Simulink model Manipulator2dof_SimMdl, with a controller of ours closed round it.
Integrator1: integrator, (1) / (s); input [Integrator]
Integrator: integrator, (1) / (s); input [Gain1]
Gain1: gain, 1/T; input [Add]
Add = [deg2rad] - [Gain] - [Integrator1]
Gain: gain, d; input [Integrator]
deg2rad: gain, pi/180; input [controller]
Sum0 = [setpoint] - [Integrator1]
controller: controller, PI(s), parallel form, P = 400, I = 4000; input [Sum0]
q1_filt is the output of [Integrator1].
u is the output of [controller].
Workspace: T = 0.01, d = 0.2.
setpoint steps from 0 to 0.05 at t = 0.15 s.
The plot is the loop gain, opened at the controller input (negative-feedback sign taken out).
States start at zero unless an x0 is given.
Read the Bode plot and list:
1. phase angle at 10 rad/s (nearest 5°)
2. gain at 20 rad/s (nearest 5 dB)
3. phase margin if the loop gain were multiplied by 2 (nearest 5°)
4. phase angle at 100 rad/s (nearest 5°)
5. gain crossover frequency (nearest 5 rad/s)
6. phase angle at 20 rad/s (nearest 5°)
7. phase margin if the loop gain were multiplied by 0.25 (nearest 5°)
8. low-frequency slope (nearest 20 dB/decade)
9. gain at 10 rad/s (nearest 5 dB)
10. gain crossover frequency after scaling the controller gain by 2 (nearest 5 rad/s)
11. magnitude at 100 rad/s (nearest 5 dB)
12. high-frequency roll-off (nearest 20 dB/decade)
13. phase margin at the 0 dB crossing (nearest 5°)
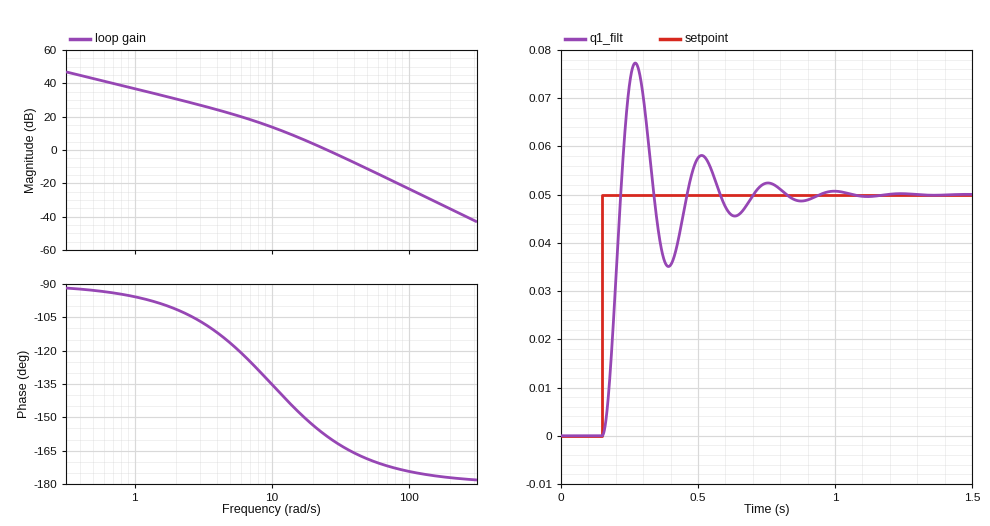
-135°
5 dB
15°
-175°
25 rad/s
-155°
40°
-20 dB/decade
15 dB
35 rad/s
-25 dB
-40 dB/decade
20°
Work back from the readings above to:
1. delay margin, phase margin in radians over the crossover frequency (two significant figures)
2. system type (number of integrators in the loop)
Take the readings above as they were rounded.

0.014 s
1
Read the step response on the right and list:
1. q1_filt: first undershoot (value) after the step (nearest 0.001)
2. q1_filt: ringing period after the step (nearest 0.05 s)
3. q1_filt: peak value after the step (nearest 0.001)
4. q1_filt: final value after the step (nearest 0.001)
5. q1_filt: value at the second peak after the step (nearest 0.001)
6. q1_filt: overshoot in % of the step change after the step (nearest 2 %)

0.035
0.25 s
0.077
0.050
0.058
54 %
